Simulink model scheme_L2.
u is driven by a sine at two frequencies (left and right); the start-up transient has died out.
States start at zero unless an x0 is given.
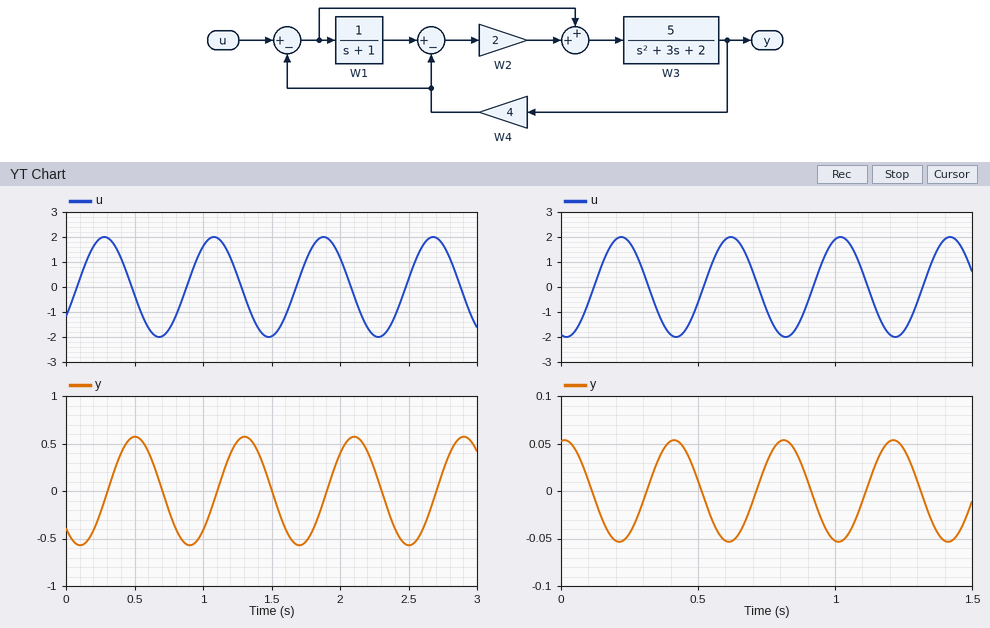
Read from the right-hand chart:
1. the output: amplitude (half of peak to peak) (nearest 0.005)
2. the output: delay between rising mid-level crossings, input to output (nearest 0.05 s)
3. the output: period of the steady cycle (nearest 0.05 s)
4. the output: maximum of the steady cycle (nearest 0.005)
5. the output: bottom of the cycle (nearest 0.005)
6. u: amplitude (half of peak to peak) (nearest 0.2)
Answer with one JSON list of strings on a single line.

["0.055", "0.20 s", "0.40 s", "0.055", "-0.055", "2.0"]
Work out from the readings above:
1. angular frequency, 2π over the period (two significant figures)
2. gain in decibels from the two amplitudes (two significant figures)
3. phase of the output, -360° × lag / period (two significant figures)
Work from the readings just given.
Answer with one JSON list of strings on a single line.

["16 rad/s", "-31 dB", "-180°"]
